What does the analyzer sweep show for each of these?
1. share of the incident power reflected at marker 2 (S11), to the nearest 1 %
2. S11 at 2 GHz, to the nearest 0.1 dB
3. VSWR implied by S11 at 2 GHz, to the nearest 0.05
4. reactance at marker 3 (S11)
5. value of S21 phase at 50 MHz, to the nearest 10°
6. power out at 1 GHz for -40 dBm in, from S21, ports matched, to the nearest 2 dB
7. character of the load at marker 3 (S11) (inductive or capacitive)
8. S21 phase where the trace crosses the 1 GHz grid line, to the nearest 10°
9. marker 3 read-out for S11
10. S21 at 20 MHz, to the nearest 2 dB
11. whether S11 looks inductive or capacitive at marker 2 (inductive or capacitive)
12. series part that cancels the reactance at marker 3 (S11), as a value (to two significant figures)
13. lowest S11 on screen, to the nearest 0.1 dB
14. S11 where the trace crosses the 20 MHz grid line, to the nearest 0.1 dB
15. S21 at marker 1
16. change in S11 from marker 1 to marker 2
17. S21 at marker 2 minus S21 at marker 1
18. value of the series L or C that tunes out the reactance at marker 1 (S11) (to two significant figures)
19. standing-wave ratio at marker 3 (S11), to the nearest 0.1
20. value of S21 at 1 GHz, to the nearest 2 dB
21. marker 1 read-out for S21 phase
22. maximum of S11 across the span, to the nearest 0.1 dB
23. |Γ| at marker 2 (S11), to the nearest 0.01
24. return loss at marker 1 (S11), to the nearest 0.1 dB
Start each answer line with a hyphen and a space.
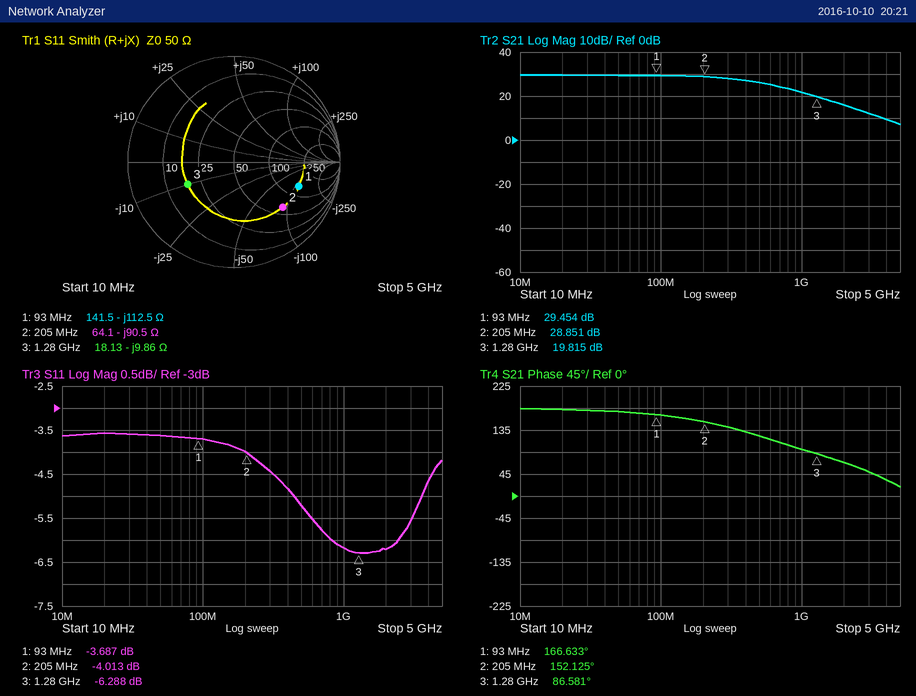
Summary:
- 40 %
- -6.2 dB
- 2.90
- -9.86 Ω
- 170°
- -18 dBm
- capacitive
- 100°
- -6.288 dB
- 30 dB
- capacitive
- 1.2 nH
- -6.3 dB
- -3.6 dB
- 29.454 dB
- -0.326 dB
- -0.603 dB
- 190 nH
- 2.9
- 22 dB
- 166.633°
- -3.6 dB
- 0.63
- 3.7 dB
